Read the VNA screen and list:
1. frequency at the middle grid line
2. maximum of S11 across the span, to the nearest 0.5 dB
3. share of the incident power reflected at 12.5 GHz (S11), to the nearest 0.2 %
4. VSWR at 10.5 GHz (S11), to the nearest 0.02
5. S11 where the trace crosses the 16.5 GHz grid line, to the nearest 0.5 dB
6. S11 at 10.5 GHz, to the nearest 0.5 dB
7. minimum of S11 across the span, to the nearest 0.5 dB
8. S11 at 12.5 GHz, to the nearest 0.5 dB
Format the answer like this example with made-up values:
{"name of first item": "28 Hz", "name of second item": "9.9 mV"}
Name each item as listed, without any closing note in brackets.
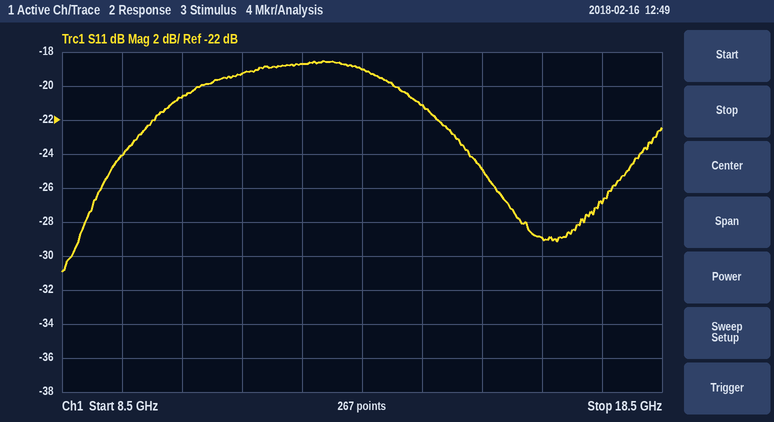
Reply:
{"frequency at the middle grid line": "13.5 GHz", "maximum of S11 across the span, to the nearest 0.5 dB": "-18.5 dB", "share of the incident power reflected at 12.5 GHz (S11), to the nearest 0.2 %": "1.4 %", "VSWR at 10.5 GHz (S11), to the nearest 0.02": "1.20", "S11 where the trace crosses the 16.5 GHz grid line, to the nearest 0.5 dB": "-29.0 dB", "S11 at 10.5 GHz, to the nearest 0.5 dB": "-20.5 dB", "minimum of S11 across the span, to the nearest 0.5 dB": "-31.0 dB", "S11 at 12.5 GHz, to the nearest 0.5 dB": "-18.5 dB"}
